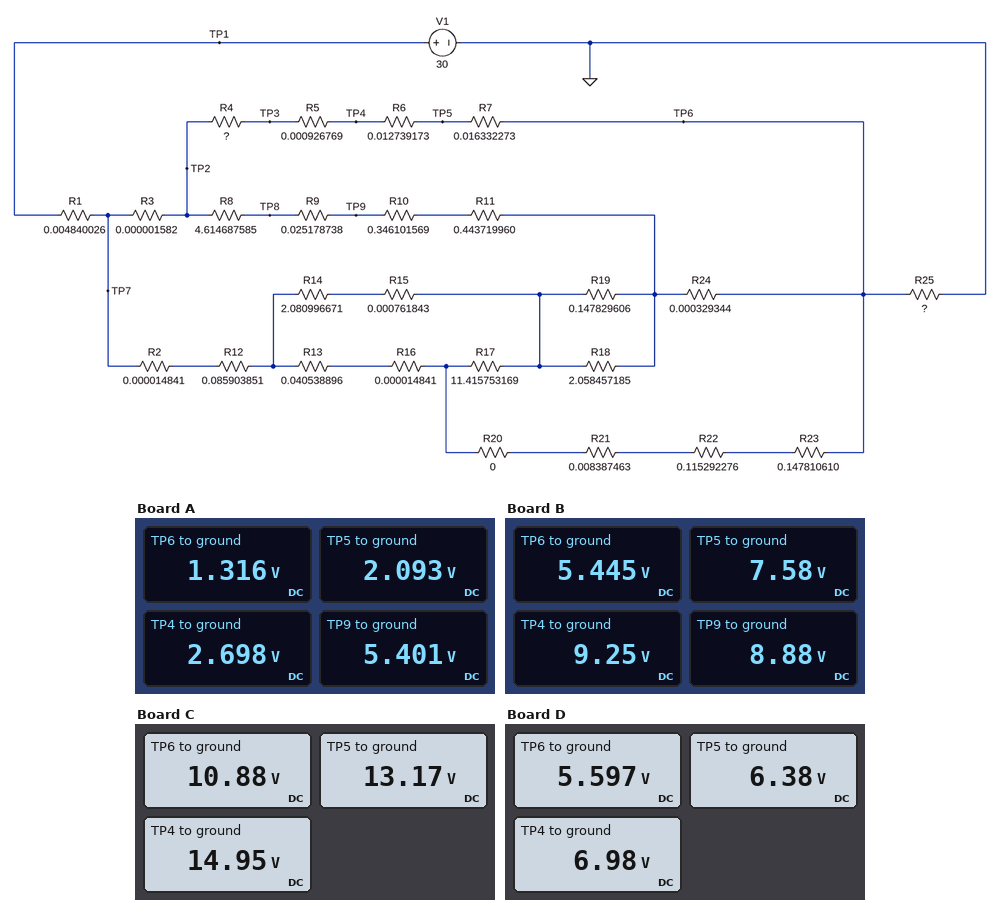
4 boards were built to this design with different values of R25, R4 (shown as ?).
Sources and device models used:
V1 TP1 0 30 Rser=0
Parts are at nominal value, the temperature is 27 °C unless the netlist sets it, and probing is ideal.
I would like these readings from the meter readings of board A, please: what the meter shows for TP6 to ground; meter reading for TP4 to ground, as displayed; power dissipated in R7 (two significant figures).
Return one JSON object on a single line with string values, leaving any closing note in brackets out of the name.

{"what the meter shows for TP6 to ground": "1.316 V", "meter reading for TP4 to ground, as displayed": "2.698 V", "power dissipated in R7": "37 W"}
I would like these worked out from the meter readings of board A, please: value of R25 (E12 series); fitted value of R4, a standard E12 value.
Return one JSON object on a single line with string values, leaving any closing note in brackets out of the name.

{"value of R25": "0.01 Ω", "fitted value of R4, a standard E12 value": "0.56 Ω"}
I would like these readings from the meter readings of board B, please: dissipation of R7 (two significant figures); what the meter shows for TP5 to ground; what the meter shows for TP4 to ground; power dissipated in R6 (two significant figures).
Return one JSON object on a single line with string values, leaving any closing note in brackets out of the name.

{"dissipation of R7": "280 W", "what the meter shows for TP5 to ground": "7.58 V", "what the meter shows for TP4 to ground": "9.25 V", "power dissipated in R6": "220 W"}
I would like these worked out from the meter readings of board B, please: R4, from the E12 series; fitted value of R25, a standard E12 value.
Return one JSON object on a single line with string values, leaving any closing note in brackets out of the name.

{"R4, from the E12 series": "0.15 Ω", "fitted value of R25, a standard E12 value": "0.027 Ω"}
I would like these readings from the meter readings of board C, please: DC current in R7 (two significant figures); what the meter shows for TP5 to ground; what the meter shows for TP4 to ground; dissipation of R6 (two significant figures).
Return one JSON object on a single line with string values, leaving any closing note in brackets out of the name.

{"DC current in R7": "140 A", "what the meter shows for TP5 to ground": "13.17 V", "what the meter shows for TP4 to ground": "14.95 V", "dissipation of R6": "250 W"}
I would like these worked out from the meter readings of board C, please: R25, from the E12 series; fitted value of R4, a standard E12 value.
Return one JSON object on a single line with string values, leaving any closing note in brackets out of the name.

{"R25, from the E12 series": "0.056 Ω", "fitted value of R4, a standard E12 value": "0.1 Ω"}
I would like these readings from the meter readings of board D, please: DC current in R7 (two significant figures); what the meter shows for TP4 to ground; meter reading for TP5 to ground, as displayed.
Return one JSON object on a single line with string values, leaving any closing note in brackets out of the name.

{"DC current in R7": "48 A", "what the meter shows for TP4 to ground": "6.98 V", "meter reading for TP5 to ground, as displayed": "6.38 V"}
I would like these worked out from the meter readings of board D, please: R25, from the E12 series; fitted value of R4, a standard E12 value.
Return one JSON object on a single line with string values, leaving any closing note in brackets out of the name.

{"R25, from the E12 series": "0.047 Ω", "fitted value of R4, a standard E12 value": "0.47 Ω"}
